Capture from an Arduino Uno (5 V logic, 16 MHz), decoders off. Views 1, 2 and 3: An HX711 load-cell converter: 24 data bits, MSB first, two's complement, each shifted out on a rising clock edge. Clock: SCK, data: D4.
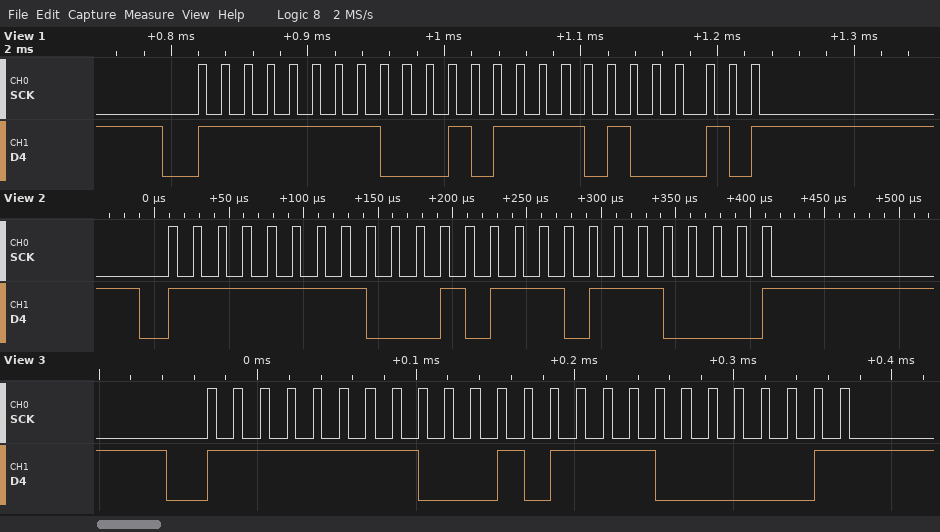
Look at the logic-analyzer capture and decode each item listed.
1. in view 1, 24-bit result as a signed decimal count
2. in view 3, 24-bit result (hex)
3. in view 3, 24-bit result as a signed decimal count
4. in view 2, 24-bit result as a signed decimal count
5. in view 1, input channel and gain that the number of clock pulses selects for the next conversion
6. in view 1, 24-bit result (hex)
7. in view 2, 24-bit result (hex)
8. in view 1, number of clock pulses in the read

-59486
0xFF1781
-59519
-59536
channel A, gain 128
0xFF17A2
0xFF1770
25
